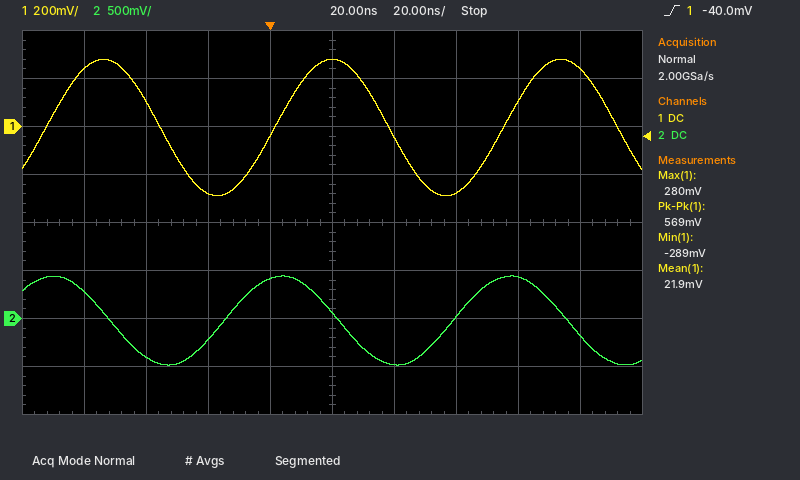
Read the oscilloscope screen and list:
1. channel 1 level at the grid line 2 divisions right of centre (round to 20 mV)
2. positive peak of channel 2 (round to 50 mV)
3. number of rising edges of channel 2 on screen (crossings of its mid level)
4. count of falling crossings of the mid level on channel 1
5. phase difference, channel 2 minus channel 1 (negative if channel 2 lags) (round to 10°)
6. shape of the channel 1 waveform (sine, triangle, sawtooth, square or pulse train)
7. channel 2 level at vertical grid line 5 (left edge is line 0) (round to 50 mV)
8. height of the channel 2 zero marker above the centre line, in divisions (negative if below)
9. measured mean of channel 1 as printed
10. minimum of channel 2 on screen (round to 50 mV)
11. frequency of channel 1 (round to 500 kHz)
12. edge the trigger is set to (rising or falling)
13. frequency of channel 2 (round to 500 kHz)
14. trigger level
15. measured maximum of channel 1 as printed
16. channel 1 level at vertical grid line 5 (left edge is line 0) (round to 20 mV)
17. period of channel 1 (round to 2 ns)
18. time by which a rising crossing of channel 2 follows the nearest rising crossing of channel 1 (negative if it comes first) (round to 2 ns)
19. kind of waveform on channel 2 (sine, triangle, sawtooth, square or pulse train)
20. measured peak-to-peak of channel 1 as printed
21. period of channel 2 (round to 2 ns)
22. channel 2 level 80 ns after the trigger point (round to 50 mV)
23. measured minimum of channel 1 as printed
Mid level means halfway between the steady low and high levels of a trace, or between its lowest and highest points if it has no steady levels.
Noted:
-280 mV
450 mV
2
3
+80°
sine
50 mV
-2.0 div
21.9 mV
-500 mV
13.5 MHz
rising
13.5 MHz
-40.0 mV
280 mV
280 mV
74 ns
-16 ns
sine
569 mV
74 ns
450 mV
-289 mV
